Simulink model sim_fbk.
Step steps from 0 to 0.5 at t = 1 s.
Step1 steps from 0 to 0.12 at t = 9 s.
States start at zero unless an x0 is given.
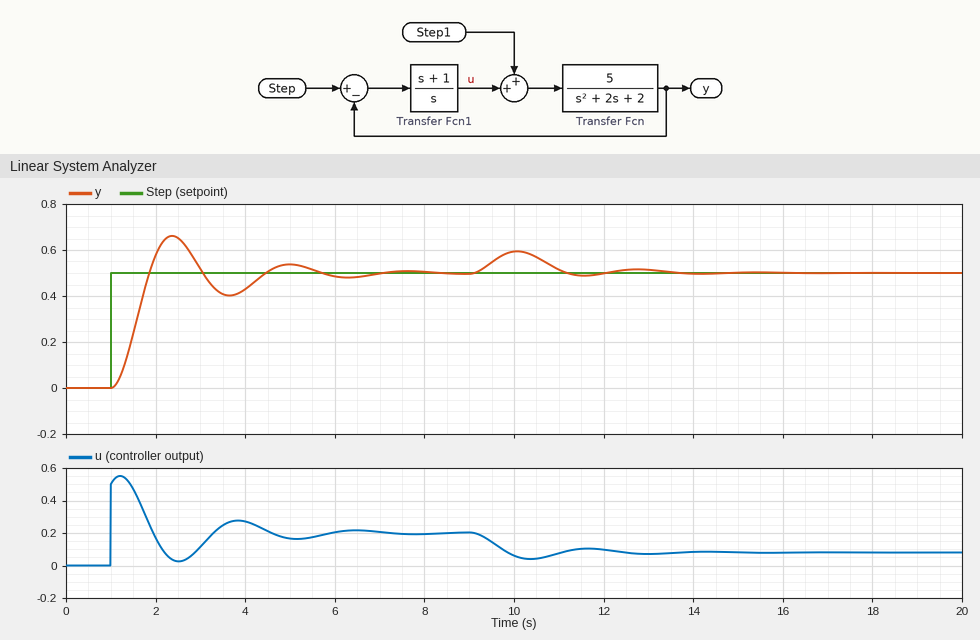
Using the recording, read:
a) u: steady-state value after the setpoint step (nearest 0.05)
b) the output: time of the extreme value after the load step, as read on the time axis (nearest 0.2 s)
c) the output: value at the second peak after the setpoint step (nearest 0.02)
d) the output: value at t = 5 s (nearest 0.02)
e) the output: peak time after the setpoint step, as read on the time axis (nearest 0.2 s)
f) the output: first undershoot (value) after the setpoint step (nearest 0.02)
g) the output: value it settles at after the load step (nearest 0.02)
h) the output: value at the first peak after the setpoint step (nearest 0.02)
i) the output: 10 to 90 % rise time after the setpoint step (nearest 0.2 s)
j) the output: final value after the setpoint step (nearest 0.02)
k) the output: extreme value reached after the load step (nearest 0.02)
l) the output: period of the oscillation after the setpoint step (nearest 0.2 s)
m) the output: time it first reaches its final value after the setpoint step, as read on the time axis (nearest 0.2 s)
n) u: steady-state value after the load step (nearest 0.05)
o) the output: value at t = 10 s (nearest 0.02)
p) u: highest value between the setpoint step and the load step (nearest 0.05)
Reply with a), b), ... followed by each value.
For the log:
a) 0.20
b) 10.0 s
c) 0.54
d) 0.54
e) 2.4 s
f) 0.40
g) 0.50
h) 0.66
i) 0.6 s
j) 0.50
k) 0.60
l) 2.6 s
m) 1.8 s
n) 0.10
o) 0.60
p) 0.55
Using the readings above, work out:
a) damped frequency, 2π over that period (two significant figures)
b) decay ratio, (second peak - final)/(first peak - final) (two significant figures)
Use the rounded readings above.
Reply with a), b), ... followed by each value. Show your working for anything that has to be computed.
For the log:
a) 2π / 2.6 = 2.4 rad/s
b) (0.54 - 0.5) / (0.66 - 0.5) = 0.25
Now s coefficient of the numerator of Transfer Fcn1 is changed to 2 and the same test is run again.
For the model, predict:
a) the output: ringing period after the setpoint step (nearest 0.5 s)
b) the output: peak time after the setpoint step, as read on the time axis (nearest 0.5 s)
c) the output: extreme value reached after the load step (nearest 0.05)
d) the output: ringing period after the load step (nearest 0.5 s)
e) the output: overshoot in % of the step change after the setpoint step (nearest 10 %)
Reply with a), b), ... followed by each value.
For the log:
a) 2.0 s
b) 2.0 s
c) 0.55
d) 2.0 s
e) 30 %
